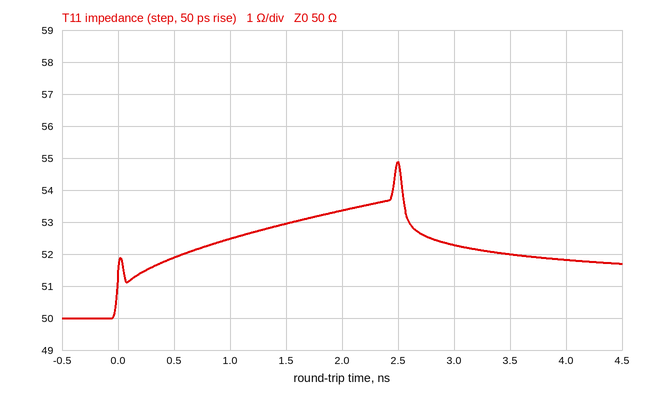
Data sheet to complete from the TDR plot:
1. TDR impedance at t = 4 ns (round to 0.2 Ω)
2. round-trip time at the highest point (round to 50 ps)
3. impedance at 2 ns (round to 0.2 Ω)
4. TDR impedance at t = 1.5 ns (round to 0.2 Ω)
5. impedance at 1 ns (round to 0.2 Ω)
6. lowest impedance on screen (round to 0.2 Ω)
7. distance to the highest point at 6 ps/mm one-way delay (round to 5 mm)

51.8 Ω
2.50 ns
53.4 Ω
53.0 Ω
52.4 Ω
50.0 Ω
210 mm
